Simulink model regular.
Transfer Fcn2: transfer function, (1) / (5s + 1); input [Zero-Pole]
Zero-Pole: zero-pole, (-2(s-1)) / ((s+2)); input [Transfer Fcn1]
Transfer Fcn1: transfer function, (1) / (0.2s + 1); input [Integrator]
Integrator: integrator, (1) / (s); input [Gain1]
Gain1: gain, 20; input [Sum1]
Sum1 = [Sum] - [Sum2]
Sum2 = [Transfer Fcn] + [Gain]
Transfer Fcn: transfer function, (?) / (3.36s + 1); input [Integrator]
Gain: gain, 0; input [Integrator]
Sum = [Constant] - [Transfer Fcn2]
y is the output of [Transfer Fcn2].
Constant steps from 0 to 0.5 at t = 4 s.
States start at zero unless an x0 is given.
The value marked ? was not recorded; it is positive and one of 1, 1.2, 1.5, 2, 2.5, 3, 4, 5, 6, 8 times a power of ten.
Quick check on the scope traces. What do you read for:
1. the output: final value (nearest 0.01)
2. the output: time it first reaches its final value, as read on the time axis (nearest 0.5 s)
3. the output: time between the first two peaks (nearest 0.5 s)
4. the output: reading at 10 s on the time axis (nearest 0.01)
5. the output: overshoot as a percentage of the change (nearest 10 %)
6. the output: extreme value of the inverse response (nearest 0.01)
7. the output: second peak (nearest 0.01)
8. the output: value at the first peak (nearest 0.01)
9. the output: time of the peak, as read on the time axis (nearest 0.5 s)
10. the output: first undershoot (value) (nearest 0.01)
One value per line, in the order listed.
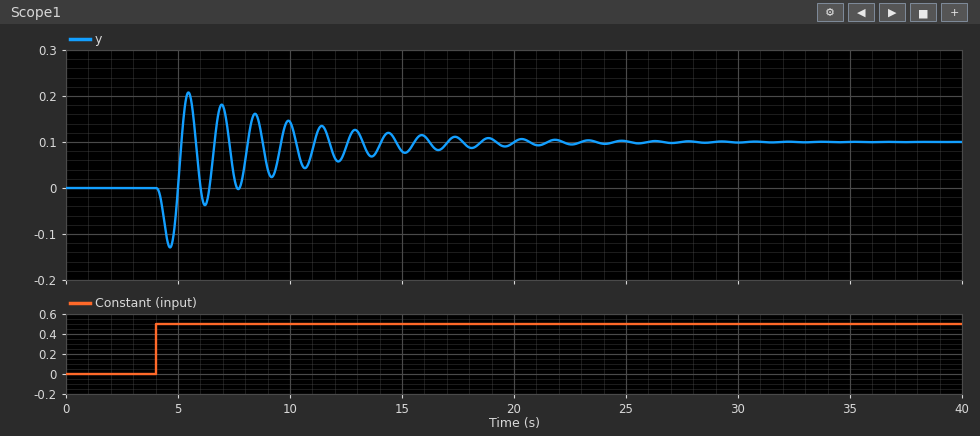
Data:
0.10
5.0 s
1.5 s
0.14
110 %
-0.13
0.18
0.21
5.5 s
-0.04
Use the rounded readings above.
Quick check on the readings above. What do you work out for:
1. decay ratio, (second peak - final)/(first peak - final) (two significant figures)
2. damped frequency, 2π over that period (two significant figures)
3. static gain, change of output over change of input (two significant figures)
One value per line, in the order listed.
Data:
0.73
4.2 rad/s
0.20
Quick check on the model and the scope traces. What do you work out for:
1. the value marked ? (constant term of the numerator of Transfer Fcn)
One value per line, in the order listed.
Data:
4
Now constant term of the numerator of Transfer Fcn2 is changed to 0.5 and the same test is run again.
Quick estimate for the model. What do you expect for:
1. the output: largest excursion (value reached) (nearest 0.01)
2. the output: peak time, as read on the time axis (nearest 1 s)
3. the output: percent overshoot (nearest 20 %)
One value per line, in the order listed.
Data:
0.09
5 s
60 %
